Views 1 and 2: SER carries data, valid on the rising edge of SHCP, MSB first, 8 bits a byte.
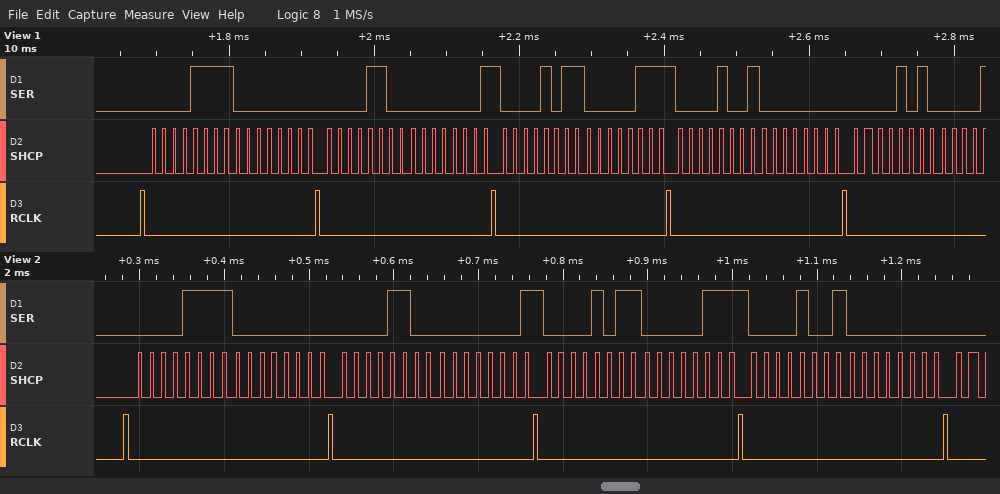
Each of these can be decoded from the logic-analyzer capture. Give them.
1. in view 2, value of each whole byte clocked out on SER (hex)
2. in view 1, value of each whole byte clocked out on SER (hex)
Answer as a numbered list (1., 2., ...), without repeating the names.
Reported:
1. 0F 00 0C 01 0B 07 09 00
2. 0x0F 0x00 0x0C 0x01 0x0B 0x07 0x09 0x00 0x0A
